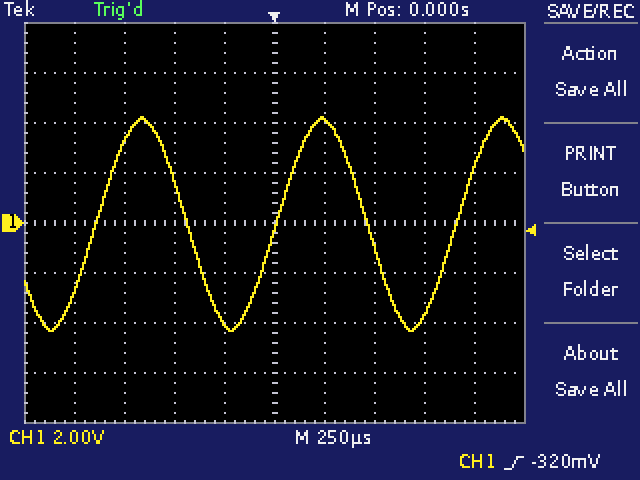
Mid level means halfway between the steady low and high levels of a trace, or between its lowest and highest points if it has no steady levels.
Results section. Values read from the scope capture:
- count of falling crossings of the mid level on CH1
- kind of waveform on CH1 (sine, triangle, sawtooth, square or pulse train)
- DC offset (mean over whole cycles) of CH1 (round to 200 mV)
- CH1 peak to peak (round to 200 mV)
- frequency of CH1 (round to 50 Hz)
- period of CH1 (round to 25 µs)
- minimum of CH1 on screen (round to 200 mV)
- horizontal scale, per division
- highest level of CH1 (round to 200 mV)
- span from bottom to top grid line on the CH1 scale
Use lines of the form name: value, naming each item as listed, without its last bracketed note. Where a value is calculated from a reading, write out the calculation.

count of falling crossings of the mid level on CH1: 2
kind of waveform on CH1: sine
DC offset (mean over whole cycles) of CH1: (4.2 V + (-4.4 V)) / 2 ≈ 0.0 V
CH1 peak to peak: 4.2 V − (-4.4 V) = 8.6 V
frequency of CH1: 1 / 900 µs ≈ 1.11 kHz, so 1.10 kHz to the nearest 50 Hz
period of CH1: 900 µs
minimum of CH1 on screen: -4.4 V
horizontal scale, per division: 250 µs
highest level of CH1: 4.2 V
span from bottom to top grid line on the CH1 scale: 16 V
